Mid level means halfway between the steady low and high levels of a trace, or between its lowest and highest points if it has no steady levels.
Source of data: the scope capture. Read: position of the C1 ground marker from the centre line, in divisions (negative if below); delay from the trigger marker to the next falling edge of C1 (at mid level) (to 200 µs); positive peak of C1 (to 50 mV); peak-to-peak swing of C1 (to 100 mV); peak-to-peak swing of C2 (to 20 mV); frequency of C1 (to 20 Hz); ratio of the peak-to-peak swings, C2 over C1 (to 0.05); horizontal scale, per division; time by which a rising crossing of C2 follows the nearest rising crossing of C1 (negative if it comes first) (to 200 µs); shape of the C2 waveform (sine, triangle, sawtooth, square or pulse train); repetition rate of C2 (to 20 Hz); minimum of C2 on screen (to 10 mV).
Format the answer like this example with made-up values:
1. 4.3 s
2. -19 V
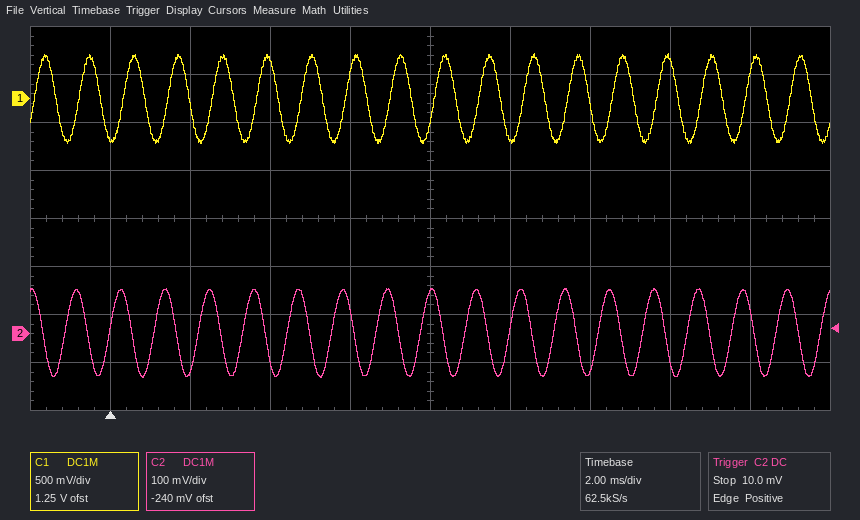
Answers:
1. +2.5 div
2. 800 µs
3. 450 mV
4. 900 mV
5. 180 mV
6. 900 Hz
7. 0.20
8. 2 ms
9. -400 µs
10. sine
11. 900 Hz
12. -90 mV
